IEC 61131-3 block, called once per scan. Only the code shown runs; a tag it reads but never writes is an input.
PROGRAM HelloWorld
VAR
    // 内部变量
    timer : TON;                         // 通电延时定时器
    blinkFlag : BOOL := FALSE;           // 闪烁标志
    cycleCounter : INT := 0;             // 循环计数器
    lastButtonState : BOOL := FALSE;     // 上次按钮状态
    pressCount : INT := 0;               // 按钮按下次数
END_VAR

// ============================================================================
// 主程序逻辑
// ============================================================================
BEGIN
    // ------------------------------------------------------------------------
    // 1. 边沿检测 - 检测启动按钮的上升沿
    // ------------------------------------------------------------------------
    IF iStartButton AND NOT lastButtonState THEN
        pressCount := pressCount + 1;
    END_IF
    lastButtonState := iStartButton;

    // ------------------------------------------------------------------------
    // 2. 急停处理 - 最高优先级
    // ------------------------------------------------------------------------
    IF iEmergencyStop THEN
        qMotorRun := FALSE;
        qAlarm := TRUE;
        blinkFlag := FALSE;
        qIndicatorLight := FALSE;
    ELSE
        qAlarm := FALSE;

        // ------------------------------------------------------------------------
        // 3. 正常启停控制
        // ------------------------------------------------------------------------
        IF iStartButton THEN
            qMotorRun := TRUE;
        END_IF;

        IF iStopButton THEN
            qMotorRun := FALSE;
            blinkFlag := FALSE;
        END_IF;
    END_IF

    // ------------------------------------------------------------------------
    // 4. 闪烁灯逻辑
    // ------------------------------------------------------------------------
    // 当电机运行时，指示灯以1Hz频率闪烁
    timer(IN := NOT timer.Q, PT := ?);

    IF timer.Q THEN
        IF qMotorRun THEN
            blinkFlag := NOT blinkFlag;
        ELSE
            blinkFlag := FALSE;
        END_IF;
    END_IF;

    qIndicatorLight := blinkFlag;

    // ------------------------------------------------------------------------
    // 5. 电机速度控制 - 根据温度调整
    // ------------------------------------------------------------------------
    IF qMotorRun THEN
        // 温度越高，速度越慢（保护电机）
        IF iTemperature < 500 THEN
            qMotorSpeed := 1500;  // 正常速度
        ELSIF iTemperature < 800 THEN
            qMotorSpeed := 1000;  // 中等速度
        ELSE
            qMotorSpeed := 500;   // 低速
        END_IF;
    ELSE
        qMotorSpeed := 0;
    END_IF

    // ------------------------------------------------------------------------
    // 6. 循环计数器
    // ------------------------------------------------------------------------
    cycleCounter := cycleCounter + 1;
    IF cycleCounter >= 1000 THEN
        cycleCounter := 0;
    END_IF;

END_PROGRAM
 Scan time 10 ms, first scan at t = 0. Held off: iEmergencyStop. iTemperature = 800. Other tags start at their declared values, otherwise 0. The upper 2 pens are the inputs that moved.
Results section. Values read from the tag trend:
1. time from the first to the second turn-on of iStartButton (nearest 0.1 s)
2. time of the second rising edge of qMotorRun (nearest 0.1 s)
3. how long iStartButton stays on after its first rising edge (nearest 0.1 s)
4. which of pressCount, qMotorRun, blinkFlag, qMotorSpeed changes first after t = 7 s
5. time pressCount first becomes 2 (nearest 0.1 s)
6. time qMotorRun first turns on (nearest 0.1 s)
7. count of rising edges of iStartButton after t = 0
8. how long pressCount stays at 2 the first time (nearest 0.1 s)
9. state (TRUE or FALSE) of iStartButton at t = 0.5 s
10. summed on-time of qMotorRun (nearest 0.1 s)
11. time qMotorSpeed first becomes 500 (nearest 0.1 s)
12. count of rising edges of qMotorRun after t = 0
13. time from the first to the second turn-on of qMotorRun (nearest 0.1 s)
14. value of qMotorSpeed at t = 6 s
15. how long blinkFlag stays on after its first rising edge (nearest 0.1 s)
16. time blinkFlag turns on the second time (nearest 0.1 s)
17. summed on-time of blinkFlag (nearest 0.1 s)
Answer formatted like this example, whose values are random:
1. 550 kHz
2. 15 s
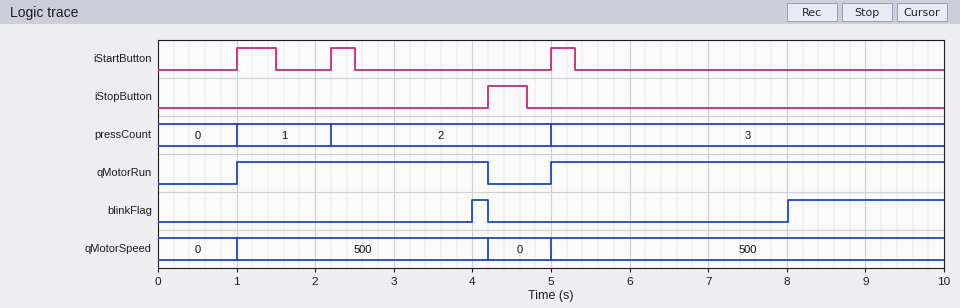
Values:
1. 1.2 s
2. 5.0 s
3. 0.5 s
4. blinkFlag
5. 2.2 s
6. 1.0 s
7. 3
8. 2.8 s
9. FALSE
10. 8.2 s
11. 1.0 s
12. 2
13. 4.0 s
14. 500
15. 0.2 s
16. 8.0 s
17. 2.2 s
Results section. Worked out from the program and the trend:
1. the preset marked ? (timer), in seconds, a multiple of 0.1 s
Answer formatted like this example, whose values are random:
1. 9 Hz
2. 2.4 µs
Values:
1. 4.0 s
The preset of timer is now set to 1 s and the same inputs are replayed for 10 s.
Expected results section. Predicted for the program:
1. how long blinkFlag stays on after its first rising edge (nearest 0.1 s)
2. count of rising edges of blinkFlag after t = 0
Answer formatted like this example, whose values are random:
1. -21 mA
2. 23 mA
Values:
1. 1.0 s
2. 5
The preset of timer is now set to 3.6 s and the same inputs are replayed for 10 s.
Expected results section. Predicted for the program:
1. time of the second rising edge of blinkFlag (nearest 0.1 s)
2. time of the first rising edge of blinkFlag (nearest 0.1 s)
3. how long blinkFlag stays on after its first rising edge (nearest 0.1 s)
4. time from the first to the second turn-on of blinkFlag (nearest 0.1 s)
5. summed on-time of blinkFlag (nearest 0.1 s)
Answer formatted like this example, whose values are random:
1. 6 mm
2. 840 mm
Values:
1. 7.2 s
2. 3.6 s
3. 0.6 s
4. 3.6 s
5. 3.4 s
